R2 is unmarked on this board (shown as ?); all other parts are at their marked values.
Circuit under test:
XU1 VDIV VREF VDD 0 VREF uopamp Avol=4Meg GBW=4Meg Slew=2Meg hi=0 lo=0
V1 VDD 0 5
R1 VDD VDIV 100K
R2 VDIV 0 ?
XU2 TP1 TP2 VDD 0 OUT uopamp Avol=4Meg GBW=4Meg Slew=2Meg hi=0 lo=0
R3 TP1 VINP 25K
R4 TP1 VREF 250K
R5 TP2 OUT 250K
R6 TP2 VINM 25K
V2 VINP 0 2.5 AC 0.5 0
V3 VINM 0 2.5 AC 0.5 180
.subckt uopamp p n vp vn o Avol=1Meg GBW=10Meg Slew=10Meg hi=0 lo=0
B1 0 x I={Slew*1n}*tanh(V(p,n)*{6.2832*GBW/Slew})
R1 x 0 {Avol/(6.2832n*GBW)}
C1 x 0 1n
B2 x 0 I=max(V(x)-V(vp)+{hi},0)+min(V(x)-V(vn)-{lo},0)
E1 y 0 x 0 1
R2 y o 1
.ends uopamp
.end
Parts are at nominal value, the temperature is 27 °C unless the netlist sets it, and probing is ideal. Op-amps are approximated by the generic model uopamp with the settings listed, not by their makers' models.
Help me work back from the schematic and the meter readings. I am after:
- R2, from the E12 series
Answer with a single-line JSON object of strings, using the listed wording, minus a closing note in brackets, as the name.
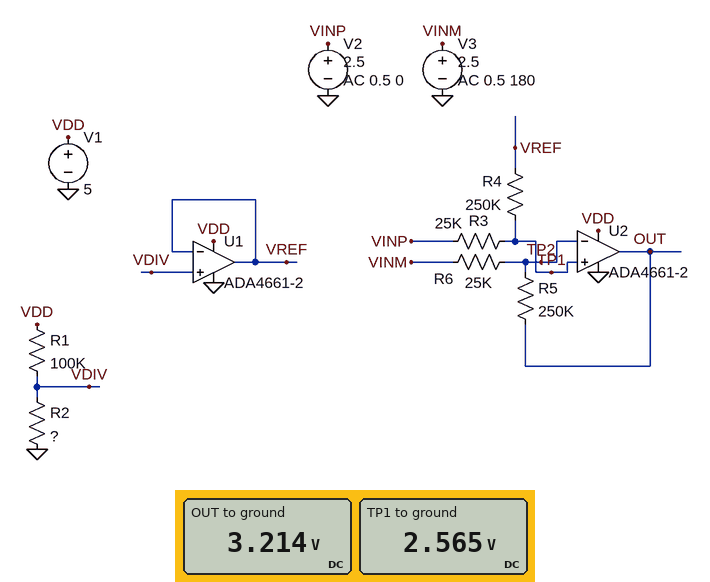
{"R2, from the E12 series": "180 kΩ"}
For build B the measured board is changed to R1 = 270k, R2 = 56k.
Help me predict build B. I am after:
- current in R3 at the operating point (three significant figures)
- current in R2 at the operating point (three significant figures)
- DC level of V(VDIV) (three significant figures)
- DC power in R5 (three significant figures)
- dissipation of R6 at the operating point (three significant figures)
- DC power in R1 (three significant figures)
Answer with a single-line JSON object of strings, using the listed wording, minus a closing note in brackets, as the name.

{"current in R3 at the operating point": "5.97 µA", "current in R2 at the operating point": "15.3 µA", "DC level of V(VDIV)": "859 mV", "DC power in R5": "8.90 µW", "dissipation of R6 at the operating point": "890 nW", "DC power in R1": "63.5 µW"}
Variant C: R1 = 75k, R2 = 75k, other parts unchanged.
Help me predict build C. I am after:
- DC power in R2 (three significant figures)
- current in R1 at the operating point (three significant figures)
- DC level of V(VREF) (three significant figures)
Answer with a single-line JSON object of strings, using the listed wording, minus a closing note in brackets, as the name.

{"DC power in R2": "83.3 µW", "current in R1 at the operating point": "33.3 µA", "DC level of V(VREF)": "2.50 V"}
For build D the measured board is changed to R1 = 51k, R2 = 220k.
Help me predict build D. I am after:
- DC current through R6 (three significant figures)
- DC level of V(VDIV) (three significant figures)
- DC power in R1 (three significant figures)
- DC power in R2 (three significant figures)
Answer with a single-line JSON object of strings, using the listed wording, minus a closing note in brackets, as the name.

{"DC current through R6": "5.67 µA", "DC level of V(VDIV)": "4.06 V", "DC power in R1": "17.4 µW", "DC power in R2": "74.9 µW"}
